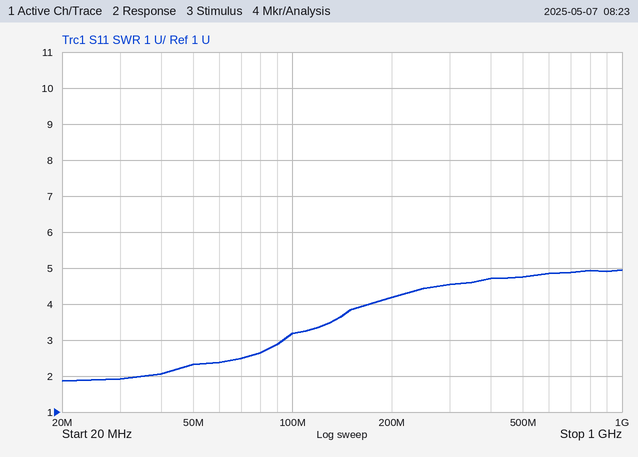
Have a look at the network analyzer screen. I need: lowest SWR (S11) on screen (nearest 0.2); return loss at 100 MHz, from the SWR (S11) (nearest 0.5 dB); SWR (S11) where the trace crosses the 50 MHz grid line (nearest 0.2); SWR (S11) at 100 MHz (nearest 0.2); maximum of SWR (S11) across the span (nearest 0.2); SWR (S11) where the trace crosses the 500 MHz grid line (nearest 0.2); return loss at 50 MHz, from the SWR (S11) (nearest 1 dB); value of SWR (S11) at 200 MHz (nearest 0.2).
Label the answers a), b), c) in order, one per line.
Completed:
a) 1.8
b) 5.5 dB
c) 2.4
d) 3.2
e) 5.0
f) 4.8
g) 8 dB
h) 4.2
